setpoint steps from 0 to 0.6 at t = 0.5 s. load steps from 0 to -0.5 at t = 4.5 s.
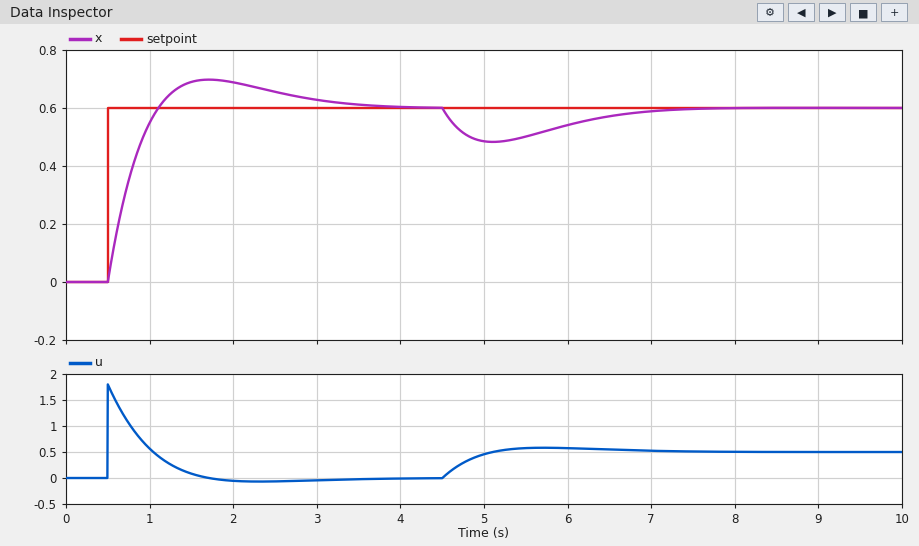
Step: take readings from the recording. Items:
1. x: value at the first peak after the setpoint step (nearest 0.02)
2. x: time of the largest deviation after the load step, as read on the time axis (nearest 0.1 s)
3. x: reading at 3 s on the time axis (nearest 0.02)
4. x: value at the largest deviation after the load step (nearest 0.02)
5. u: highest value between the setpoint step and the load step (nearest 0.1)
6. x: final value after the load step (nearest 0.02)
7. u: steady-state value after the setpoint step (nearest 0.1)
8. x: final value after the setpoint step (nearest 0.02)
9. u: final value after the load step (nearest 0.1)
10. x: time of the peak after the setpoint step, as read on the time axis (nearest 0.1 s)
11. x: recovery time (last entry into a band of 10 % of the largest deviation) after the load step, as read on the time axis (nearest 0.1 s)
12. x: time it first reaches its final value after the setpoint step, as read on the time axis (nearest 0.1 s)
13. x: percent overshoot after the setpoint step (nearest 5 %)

0.70
5.1 s
0.62
0.48
1.8
0.60
0.0
0.60
0.5
1.7 s
7.0 s
1.1 s
15 %
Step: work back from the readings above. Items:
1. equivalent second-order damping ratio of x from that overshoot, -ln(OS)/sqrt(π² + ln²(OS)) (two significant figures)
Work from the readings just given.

0.52
